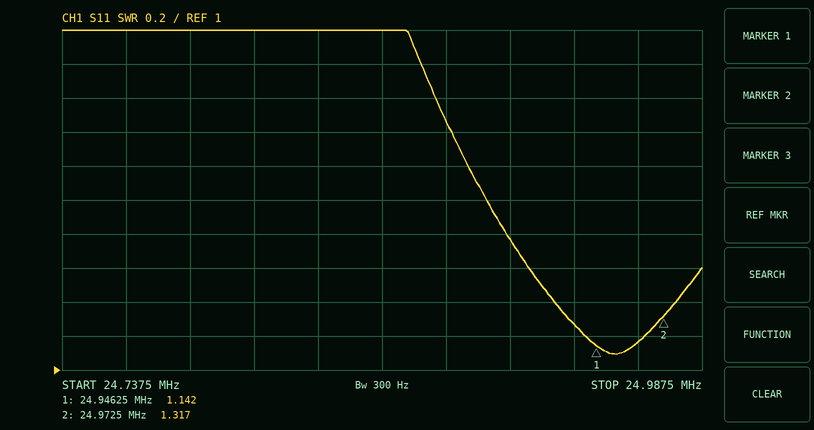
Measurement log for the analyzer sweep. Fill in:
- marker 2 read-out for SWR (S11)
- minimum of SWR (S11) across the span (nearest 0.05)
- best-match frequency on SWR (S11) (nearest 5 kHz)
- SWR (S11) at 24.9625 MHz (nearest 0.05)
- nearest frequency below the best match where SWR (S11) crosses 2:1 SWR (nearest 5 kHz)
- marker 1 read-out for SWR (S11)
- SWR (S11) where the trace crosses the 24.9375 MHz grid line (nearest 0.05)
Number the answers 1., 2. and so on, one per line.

1. 1.317
2. 1.10
3. 24.955 MHz
4. 1.15
5. 24.905 MHz
6. 1.142
7. 1.25
